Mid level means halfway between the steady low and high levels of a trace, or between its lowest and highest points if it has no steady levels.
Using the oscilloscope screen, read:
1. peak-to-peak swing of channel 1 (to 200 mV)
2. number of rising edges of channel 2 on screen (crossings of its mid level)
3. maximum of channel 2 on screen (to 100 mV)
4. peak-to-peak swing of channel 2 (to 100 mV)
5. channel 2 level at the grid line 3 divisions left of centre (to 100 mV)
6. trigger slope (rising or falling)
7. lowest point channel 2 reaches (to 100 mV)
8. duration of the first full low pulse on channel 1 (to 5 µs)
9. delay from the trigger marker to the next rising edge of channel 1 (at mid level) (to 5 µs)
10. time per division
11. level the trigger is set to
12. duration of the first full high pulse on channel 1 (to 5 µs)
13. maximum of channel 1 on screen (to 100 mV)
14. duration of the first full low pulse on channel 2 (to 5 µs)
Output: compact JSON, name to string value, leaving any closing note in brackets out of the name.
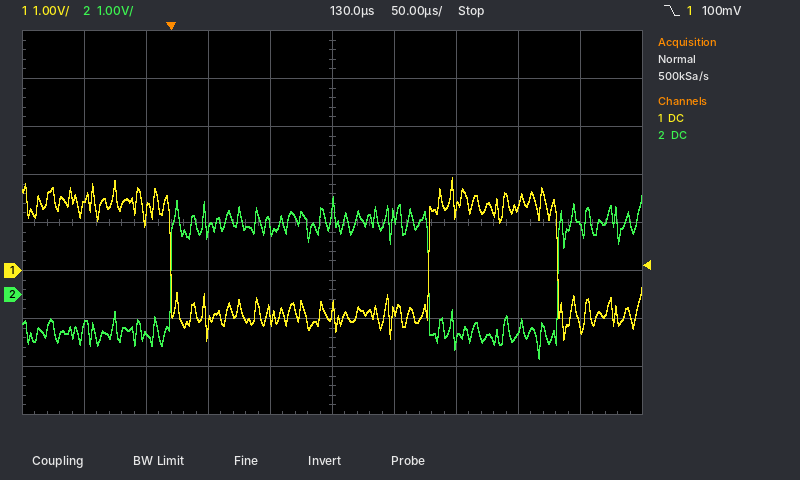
{"peak-to-peak swing of channel 1": "3.4 V", "number of rising edges of channel 2 on screen": "2", "maximum of channel 2 on screen": "2.1 V", "peak-to-peak swing of channel 2": "3.4 V", "channel 2 level at the grid line 3 divisions left of centre": "-800 mV", "trigger slope": "falling", "lowest point channel 2 reaches": "-1.3 V", "duration of the first full low pulse on channel 1": "210 µs", "delay from the trigger marker to the next rising edge of channel 1 (at mid level)": "210 µs", "time per division": "50 µs", "level the trigger is set to": "100 mV", "duration of the first full high pulse on channel 1": "105 µs", "maximum of channel 1 on screen": "1.9 V", "duration of the first full low pulse on channel 2": "105 µs"}
